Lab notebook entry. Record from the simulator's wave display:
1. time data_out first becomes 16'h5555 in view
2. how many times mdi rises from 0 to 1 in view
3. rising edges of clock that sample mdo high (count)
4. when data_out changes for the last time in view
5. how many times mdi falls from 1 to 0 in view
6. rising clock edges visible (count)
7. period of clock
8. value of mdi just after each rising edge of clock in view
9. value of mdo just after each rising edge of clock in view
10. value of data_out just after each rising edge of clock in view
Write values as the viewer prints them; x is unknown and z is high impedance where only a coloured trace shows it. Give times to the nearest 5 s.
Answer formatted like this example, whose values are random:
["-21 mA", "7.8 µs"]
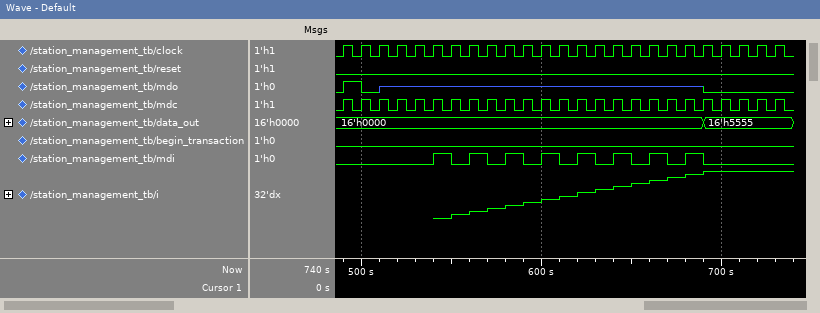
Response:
["690 s", "8", "1", "690 s", "8", "25", "10 s", "0 0 0 0 0 1 0 1 0 1 0 1 0 1 0 1 0 1 0 1 0 0 0 0 0", "1 0 z z z z z z z z z z z z z z z z z z 0 0 0 0 0", "16'h0000, 16'h0000, 16'h0000, 16'h0000, 16'h0000, 16'h0000, 16'h0000, 16'h0000, 16'h0000, 16'h0000, 16'h0000, 16'h0000, 16'h0000, 16'h0000, 16'h0000, 16'h0000, 16'h0000, 16'h0000, 16'h0000, 16'h0000, 16'h5555, 16'h5555, 16'h5555, 16'h5555, 16'h5555"]
